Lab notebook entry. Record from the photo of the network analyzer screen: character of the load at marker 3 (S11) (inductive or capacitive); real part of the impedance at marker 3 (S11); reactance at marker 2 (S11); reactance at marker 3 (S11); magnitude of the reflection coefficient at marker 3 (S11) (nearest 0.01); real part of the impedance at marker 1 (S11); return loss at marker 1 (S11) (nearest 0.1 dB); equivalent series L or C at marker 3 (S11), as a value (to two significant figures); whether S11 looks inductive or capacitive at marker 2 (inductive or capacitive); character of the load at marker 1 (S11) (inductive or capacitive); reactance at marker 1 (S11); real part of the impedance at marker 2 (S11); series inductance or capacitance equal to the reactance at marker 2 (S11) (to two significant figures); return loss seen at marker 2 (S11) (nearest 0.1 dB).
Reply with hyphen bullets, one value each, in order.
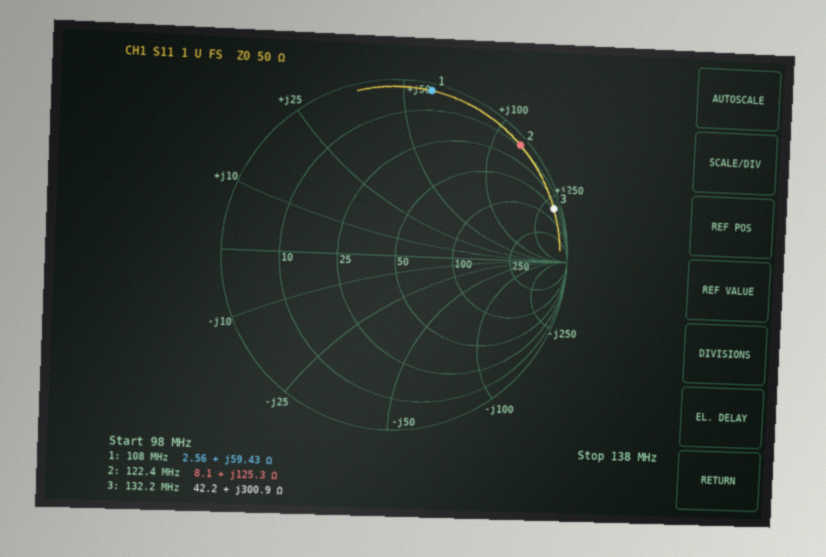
- inductive
- 42.2 Ω
- +125.3 Ω
- +300.9 Ω
- 0.96
- 2.56 Ω
- 0.4 dB
- 360 nH
- inductive
- inductive
- +59.43 Ω
- 8.1 Ω
- 160 nH
- 0.4 dB
